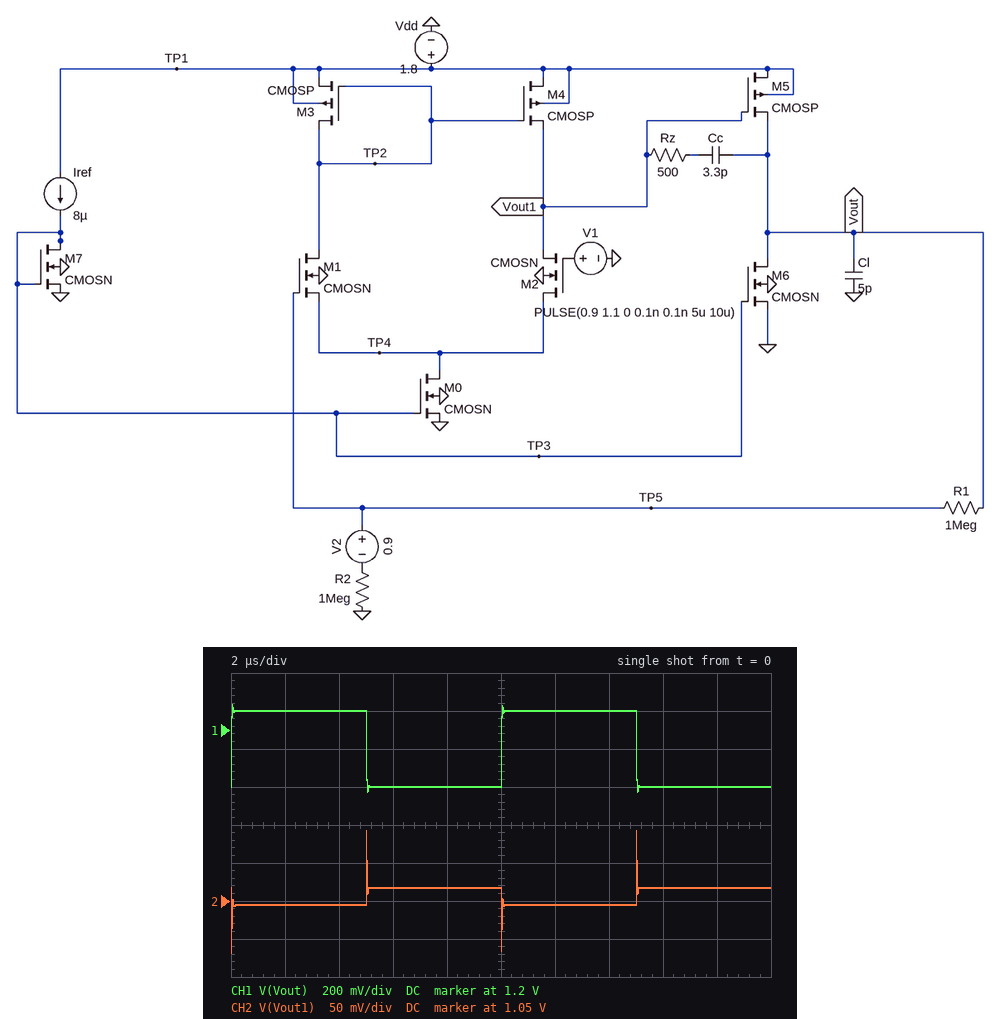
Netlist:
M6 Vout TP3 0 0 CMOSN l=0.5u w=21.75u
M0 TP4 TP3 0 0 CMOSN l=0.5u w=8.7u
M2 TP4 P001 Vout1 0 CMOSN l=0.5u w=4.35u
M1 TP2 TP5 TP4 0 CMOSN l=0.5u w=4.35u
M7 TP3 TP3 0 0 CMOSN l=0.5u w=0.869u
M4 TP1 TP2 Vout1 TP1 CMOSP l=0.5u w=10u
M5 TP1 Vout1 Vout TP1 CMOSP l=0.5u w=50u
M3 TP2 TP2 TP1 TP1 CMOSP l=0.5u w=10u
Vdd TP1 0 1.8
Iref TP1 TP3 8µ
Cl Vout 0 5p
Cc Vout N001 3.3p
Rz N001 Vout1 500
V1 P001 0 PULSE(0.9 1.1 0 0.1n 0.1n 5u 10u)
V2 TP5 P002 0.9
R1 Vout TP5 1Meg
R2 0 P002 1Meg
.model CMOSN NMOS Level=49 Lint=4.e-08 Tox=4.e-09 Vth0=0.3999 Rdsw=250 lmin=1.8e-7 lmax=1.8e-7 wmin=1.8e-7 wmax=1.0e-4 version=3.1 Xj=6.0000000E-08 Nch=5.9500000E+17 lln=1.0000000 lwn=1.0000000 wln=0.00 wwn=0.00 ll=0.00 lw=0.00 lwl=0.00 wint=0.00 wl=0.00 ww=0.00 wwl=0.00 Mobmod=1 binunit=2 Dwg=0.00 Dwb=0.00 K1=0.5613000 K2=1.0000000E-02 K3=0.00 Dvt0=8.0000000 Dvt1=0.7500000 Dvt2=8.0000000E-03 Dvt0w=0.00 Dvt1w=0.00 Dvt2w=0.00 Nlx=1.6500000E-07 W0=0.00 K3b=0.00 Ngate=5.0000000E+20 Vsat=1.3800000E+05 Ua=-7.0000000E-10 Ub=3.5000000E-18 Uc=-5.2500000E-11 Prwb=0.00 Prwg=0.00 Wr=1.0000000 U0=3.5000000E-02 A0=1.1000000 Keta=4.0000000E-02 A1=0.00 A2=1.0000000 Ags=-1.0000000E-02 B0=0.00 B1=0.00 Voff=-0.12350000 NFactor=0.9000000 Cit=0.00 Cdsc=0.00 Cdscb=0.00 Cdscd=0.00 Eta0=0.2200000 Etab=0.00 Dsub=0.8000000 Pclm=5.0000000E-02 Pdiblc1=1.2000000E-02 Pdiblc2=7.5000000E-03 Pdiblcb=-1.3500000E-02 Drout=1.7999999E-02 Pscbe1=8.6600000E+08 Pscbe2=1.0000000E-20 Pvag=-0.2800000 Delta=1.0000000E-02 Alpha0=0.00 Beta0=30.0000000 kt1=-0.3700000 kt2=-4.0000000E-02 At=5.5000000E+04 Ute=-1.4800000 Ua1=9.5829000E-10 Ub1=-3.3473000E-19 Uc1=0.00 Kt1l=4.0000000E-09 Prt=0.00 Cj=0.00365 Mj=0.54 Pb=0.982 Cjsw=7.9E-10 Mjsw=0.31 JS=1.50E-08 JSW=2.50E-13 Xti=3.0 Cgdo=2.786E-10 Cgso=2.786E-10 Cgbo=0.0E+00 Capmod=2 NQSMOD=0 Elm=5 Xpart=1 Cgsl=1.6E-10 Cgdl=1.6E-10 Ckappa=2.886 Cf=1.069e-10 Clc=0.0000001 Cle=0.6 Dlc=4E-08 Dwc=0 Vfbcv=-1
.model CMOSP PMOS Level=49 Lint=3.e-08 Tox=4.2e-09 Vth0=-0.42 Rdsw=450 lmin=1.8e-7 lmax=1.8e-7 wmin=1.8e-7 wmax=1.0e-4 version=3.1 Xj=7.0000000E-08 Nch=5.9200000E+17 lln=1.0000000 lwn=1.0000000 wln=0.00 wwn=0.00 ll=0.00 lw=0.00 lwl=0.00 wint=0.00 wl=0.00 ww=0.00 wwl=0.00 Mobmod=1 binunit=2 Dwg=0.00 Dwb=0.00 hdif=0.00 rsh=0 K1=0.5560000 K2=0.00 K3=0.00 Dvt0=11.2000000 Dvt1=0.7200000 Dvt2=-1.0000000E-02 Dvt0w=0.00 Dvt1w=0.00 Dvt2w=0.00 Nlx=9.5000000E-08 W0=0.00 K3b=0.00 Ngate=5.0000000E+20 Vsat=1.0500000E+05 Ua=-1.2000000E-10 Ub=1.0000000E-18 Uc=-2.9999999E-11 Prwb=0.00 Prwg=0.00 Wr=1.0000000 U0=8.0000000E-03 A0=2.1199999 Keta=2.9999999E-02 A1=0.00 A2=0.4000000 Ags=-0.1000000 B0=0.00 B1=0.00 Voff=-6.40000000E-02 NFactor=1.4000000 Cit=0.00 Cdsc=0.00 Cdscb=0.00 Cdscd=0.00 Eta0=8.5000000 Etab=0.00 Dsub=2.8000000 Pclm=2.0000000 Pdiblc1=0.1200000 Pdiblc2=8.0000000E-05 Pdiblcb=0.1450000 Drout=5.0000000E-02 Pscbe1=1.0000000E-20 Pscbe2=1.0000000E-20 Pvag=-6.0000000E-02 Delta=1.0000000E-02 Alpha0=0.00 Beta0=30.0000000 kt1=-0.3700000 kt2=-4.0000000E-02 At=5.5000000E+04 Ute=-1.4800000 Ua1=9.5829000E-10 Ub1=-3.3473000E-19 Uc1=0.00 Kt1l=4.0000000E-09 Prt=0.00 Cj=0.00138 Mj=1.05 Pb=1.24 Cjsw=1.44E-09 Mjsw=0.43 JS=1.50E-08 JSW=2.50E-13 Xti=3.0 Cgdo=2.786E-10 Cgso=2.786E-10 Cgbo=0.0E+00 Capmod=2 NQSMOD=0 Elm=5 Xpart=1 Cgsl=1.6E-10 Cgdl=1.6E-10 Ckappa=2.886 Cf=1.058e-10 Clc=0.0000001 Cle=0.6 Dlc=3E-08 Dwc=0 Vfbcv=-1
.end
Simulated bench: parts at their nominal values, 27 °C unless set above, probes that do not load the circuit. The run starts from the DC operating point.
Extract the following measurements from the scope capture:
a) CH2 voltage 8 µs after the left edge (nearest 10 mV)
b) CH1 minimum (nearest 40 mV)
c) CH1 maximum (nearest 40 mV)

1.07 V
880 mV
1.32 V
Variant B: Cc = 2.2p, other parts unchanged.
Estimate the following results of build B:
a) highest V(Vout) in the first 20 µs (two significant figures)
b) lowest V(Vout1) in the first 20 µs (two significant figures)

1.4 V
960 mV
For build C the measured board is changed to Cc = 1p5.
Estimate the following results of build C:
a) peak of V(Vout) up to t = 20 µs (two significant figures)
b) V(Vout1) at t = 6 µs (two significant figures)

1.4 V
1.1 V
